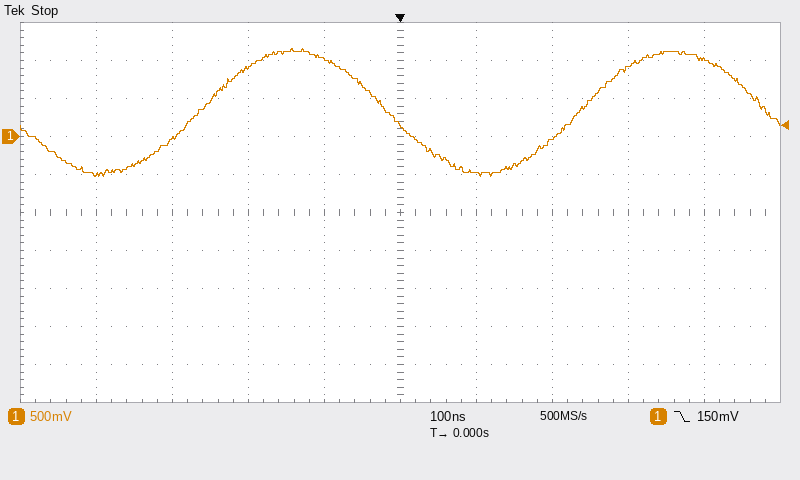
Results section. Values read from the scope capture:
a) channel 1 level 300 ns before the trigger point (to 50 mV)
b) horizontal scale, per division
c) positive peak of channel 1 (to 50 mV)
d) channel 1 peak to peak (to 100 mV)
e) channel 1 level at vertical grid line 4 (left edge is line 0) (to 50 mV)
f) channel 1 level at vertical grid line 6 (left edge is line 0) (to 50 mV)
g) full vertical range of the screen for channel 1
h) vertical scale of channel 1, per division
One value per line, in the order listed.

-50 mV
100 ns
1.15 V
1.70 V
1.00 V
-500 mV
5 V
500 mV
